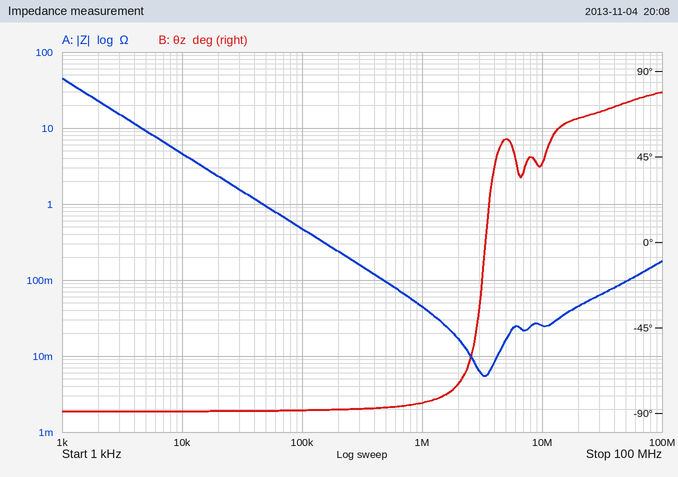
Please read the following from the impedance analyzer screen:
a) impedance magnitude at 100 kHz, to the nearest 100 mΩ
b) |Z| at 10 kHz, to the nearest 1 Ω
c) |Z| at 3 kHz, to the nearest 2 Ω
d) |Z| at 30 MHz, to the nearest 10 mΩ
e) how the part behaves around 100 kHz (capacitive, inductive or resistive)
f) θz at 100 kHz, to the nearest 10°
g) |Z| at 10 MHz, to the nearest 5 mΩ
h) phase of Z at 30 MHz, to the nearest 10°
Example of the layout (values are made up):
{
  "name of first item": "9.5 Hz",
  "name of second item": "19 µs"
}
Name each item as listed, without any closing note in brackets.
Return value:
{
  "impedance magnitude at 100 kHz, to the nearest 100 mΩ": "500 mΩ",
  "|Z| at 10 kHz, to the nearest 1 Ω": "5 Ω",
  "|Z| at 3 kHz, to the nearest 2 Ω": "16 Ω",
  "|Z| at 30 MHz, to the nearest 10 mΩ": "60 mΩ",
  "how the part behaves around 100 kHz": "capacitive",
  "θz at 100 kHz, to the nearest 10°": "-90°",
  "|Z| at 10 MHz, to the nearest 5 mΩ": "25 mΩ",
  "phase of Z at 30 MHz, to the nearest 10°": "70°"
}
